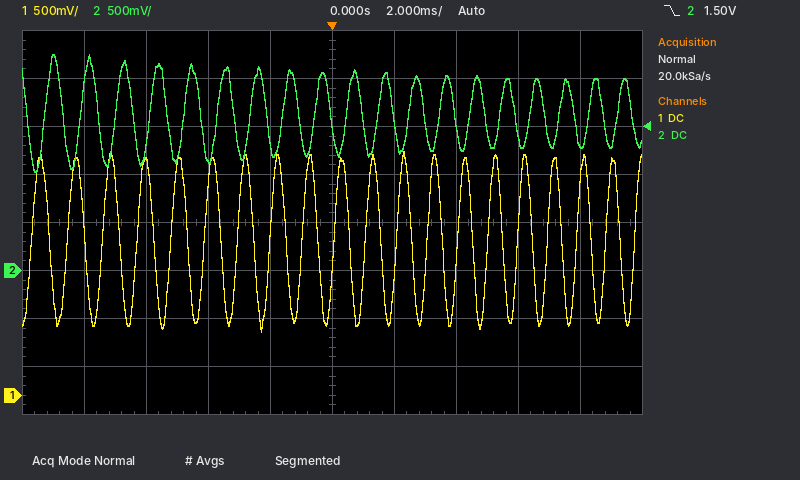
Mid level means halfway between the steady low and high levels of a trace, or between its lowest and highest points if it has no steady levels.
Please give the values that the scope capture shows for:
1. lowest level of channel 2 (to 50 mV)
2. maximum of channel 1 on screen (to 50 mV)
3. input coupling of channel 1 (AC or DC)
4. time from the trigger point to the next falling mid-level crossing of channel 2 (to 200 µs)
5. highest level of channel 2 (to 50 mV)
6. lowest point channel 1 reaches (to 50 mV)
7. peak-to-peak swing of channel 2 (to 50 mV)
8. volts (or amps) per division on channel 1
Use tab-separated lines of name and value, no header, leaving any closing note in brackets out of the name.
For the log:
lowest level of channel 2	1.05 V
maximum of channel 1 on screen	2.55 V
input coupling of channel 1	DC
time from the trigger point to the next falling mid-level crossing of channel 2	1.0 ms
highest level of channel 2	2.25 V
lowest point channel 1 reaches	650 mV
peak-to-peak swing of channel 2	1.20 V
volts (or amps) per division on channel 1	500 mV
